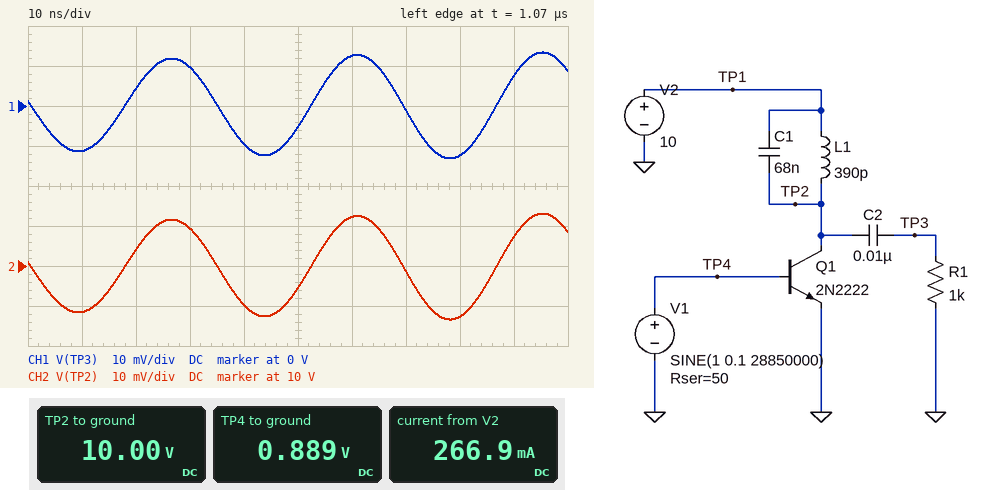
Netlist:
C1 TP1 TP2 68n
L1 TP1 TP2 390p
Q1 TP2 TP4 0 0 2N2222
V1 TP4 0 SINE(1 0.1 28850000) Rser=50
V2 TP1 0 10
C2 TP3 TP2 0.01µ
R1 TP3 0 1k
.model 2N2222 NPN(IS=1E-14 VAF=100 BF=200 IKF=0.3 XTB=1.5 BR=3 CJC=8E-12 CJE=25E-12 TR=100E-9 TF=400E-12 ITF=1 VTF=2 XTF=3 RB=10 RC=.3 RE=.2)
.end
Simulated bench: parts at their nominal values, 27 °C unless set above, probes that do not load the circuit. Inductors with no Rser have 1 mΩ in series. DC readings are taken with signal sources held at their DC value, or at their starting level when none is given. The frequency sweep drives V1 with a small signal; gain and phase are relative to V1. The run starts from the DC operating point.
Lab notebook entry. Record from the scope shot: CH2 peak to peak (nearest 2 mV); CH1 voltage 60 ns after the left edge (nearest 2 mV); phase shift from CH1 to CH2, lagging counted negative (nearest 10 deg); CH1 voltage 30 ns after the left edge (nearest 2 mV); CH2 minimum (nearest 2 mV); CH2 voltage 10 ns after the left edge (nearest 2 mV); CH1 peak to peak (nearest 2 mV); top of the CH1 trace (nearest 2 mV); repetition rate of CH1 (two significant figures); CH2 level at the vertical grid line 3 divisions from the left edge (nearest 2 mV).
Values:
26 mV
12 mV
0 deg
10 mV
9.986 V
9.988 V
26 mV
14 mV
29 MHz
10.010 V
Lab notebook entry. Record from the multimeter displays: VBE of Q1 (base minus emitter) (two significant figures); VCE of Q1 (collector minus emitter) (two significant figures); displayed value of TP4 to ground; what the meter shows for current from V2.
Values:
890 mV
10 V
0.889 V
266.9 mA
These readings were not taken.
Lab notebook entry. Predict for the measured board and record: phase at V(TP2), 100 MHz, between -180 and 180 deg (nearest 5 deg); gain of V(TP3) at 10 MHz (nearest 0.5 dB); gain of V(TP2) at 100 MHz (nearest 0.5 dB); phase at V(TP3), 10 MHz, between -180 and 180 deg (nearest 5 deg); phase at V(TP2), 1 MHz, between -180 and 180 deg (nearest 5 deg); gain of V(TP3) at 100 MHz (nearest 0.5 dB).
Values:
5 deg
-37.0 dB
-56.0 dB
-150 deg
-120 deg
-56.0 dB
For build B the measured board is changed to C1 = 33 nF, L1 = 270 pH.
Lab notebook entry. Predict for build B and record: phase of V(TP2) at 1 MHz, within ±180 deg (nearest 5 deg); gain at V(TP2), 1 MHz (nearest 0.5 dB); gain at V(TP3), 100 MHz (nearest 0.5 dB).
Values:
-130 deg
-55.0 dB
-47.5 dB
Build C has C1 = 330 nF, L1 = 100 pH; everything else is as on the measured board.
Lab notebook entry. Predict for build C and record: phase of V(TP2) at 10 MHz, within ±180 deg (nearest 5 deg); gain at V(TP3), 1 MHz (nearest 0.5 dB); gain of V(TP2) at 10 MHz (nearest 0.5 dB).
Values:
-155 deg
-59.0 dB
-48.5 dB
